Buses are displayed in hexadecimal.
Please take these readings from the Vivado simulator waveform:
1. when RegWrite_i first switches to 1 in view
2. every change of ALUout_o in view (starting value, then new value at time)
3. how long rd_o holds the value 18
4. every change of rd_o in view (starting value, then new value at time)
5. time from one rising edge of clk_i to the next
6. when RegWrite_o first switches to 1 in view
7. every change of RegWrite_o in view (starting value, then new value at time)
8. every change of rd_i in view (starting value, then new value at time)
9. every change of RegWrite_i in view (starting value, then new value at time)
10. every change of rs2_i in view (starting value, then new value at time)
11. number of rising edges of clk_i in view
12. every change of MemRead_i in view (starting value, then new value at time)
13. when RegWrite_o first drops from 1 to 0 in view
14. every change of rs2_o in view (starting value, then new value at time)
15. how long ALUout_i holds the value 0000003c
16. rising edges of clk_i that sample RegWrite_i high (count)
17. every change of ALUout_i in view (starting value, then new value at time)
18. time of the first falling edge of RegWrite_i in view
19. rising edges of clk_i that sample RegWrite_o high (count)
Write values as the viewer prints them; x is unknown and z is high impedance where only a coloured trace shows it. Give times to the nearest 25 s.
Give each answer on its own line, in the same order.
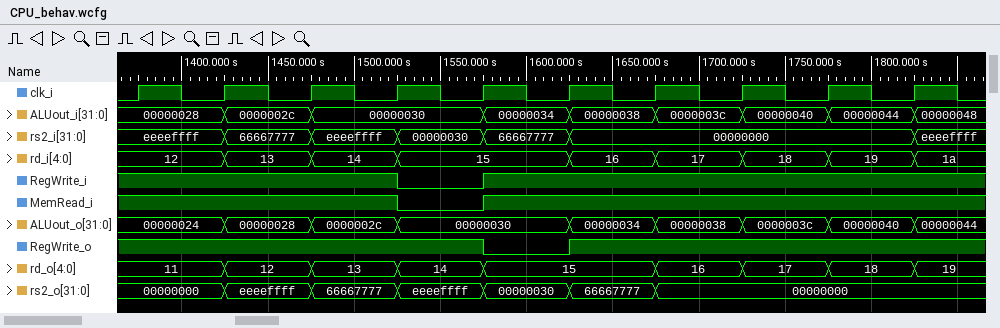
1575 s
00000024, 00000028 at 1425 s, 0000002c at 1475 s, 00000030 at 1525 s, 00000034 at 1625 s, 00000038 at 1675 s, 0000003c at 1725 s, 00000040 at 1775 s, 00000044 at 1825 s
50 s
11, 12 at 1425 s, 13 at 1475 s, 14 at 1525 s, 15 at 1575 s, 16 at 1675 s, 17 at 1725 s, 18 at 1775 s, 19 at 1825 s
50 s
1625 s
1, 0 at 1575 s, 1 at 1625 s
12, 13 at 1425 s, 14 at 1475 s, 15 at 1525 s, 16 at 1625 s, 17 at 1675 s, 18 at 1725 s, 19 at 1775 s, 1a at 1825 s
1, 0 at 1525 s, 1 at 1575 s
eeeeffff, 66667777 at 1425 s, eeeeffff at 1475 s, 00000030 at 1525 s, 66667777 at 1575 s, 00000000 at 1625 s, eeeeffff at 1825 s
10
1, 0 at 1525 s, 1 at 1575 s
1575 s
00000000, eeeeffff at 1425 s, 66667777 at 1475 s, eeeeffff at 1525 s, 00000030 at 1575 s, 66667777 at 1625 s, 00000000 at 1675 s
50 s
9
00000028, 0000002c at 1425 s, 00000030 at 1475 s, 00000034 at 1575 s, 00000038 at 1625 s, 0000003c at 1675 s, 00000040 at 1725 s, 00000044 at 1775 s, 00000048 at 1825 s
1525 s
9
